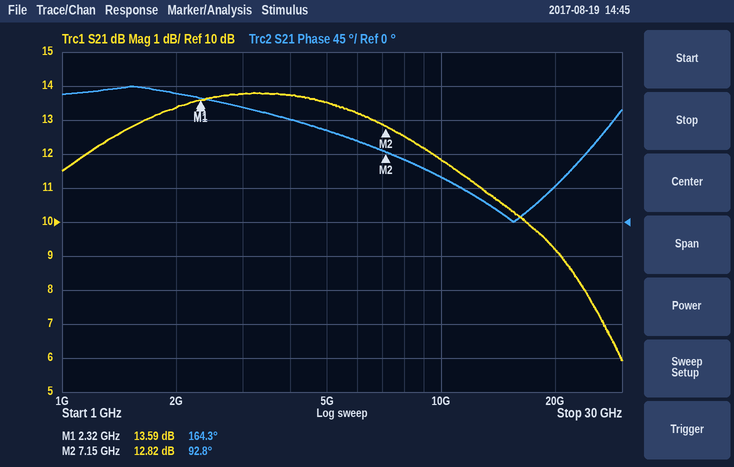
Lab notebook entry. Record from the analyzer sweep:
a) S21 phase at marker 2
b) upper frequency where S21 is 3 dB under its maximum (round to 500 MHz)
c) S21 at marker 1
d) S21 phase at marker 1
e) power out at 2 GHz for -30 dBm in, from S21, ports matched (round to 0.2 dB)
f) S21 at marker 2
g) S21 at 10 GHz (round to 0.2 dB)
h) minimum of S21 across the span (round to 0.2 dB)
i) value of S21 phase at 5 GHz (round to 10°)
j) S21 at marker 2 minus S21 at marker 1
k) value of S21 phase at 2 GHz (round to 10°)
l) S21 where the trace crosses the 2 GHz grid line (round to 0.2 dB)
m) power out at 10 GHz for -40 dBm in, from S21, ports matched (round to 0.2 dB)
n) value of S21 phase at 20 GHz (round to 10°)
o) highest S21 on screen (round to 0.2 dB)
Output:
92.8°
13.5 GHz
13.59 dB
164.3°
-16.6 dBm
12.82 dB
11.8 dB
6.0 dB
120°
-0.77 dB
170°
13.4 dB
-28.2 dBm
50°
13.8 dB
